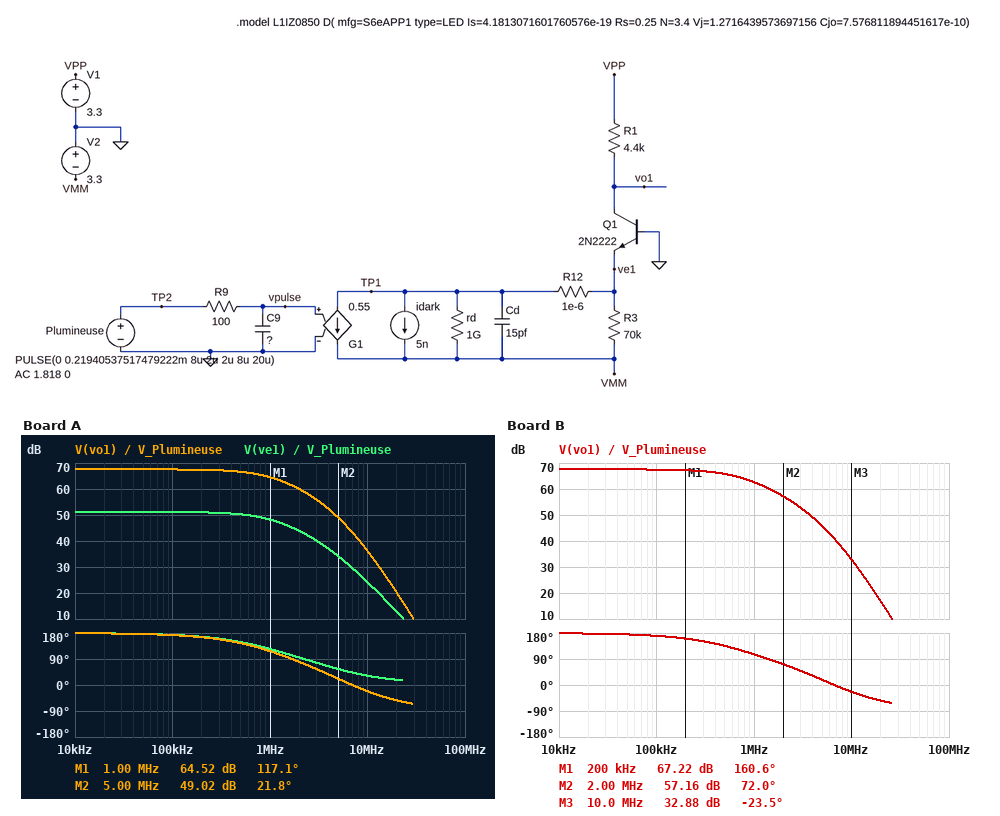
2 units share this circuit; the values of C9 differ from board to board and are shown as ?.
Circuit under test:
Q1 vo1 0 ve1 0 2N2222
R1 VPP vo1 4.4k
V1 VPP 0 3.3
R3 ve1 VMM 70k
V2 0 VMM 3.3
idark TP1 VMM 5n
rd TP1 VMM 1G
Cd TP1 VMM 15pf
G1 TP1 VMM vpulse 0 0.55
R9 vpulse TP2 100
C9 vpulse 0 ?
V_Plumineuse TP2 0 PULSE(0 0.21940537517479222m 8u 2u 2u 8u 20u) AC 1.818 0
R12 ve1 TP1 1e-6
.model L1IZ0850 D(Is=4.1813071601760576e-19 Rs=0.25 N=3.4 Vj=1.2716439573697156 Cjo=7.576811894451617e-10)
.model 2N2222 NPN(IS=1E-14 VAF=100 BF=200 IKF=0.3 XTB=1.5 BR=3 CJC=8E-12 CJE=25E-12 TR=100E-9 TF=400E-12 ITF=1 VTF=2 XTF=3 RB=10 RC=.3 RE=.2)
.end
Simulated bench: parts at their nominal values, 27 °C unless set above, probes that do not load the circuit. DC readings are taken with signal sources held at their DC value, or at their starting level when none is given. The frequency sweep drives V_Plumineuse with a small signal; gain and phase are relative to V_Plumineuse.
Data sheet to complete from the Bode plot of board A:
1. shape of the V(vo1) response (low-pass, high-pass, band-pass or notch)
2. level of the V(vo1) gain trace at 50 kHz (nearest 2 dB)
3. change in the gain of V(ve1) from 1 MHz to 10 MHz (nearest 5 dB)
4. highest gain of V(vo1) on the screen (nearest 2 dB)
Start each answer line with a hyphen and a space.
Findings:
- low-pass
- 68 dB
- -25 dB
- 68 dB
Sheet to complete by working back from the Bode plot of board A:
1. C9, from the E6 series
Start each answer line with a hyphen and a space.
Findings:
- 1.5 nF
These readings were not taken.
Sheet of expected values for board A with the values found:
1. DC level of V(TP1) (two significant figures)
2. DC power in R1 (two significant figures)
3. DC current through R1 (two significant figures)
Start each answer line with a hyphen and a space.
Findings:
- -570 mV
- 6.6 µW
- 39 µA
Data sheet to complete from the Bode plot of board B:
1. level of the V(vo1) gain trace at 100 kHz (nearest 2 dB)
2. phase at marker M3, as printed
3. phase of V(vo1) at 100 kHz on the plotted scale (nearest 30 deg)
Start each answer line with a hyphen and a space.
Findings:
- 68 dB
- -23.5 deg
- 180 deg
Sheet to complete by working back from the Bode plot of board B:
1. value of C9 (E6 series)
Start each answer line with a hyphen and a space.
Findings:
- 2.2 nF
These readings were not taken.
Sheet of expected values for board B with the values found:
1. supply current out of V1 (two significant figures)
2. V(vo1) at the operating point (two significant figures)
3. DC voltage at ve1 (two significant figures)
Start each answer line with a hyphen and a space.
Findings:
- 39 µA
- 3.1 V
- -570 mV
